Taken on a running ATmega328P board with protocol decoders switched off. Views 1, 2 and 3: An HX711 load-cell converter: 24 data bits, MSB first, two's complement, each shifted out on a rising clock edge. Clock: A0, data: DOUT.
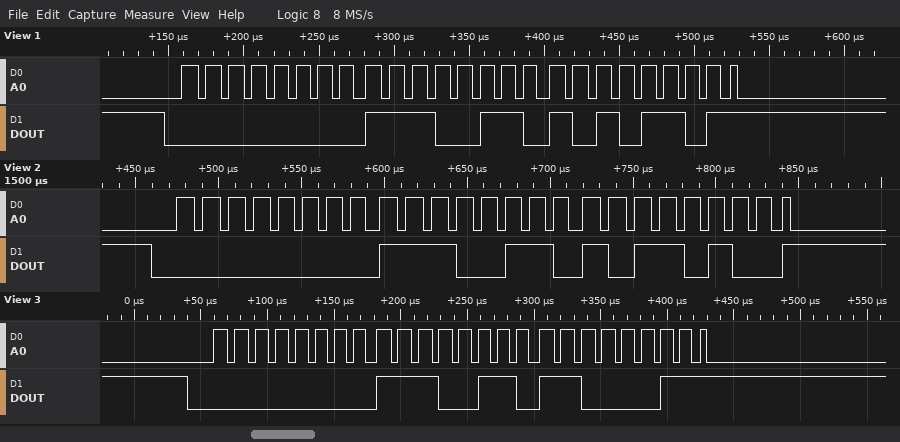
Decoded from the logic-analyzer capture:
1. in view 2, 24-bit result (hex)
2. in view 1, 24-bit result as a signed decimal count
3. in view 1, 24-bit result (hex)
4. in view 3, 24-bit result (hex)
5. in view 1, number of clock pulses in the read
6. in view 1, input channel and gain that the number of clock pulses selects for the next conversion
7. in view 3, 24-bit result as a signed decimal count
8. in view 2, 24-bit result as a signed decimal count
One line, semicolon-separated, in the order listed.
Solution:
0x00E6B4; 59053; 0x00E6AD; 0x00E6C3; 25; channel A, gain 128; 59075; 59060
